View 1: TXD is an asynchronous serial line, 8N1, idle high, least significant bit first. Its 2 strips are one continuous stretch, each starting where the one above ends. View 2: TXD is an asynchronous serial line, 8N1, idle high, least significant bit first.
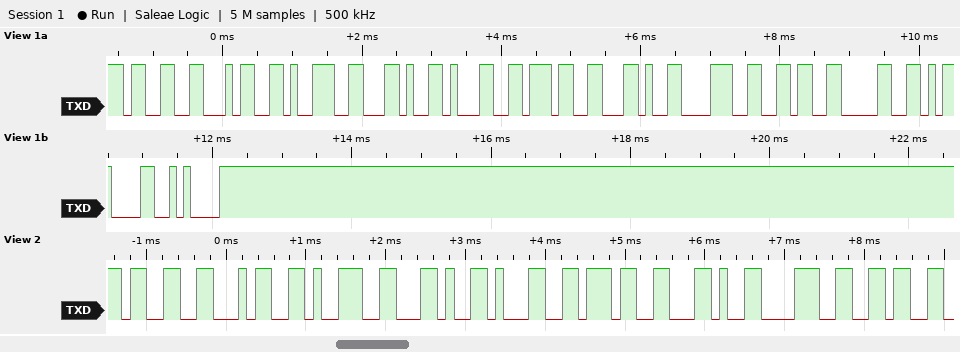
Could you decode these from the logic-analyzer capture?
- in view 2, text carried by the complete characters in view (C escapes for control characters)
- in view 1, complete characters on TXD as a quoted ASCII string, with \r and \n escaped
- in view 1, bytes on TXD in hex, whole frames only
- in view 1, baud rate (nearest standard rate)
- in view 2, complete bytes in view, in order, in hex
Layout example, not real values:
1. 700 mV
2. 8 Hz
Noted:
1. "349,17,86"
2. "349,17,860\r\n"
3. 0x33 0x34 0x39 0x2C 0x31 0x37 0x2C 0x38 0x36 0x30 0x0D 0x0A
4. 9600 baud
5. 33 34 39 2C 31 37 2C 38 36
